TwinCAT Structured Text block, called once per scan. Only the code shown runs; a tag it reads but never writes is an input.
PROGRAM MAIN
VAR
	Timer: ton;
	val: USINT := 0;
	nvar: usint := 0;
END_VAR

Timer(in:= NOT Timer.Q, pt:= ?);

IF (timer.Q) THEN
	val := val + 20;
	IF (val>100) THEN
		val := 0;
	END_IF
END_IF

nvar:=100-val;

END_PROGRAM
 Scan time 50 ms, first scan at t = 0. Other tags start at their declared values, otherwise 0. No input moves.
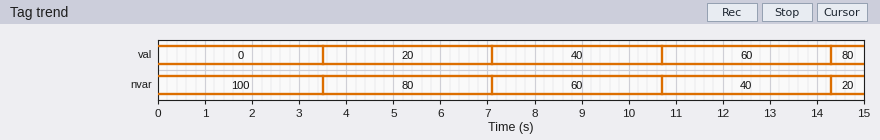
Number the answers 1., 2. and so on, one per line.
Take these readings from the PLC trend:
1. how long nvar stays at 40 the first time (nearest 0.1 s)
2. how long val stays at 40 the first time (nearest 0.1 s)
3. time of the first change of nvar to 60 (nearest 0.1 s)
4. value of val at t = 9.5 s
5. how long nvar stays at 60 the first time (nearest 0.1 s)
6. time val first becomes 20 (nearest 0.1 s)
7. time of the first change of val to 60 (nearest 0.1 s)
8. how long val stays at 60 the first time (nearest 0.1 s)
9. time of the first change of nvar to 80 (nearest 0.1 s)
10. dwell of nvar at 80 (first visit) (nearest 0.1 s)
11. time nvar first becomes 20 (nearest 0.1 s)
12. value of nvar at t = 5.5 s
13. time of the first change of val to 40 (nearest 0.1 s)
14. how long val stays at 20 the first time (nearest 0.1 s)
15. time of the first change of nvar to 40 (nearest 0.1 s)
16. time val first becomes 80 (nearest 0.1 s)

1. 3.6 s
2. 3.6 s
3. 7.1 s
4. 40
5. 3.6 s
6. 3.5 s
7. 10.7 s
8. 3.6 s
9. 3.5 s
10. 3.6 s
11. 14.3 s
12. 80
13. 7.1 s
14. 3.6 s
15. 10.7 s
16. 14.3 s
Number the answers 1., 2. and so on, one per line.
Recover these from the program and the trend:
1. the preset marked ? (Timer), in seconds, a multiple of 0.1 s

1. 3.5 s
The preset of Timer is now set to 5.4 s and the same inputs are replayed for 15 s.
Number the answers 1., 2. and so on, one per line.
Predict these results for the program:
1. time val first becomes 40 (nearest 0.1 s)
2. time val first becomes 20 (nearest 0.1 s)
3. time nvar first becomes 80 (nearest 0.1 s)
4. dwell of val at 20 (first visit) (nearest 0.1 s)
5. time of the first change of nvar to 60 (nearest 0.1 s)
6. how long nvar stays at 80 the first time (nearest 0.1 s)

1. 10.9 s
2. 5.4 s
3. 5.4 s
4. 5.5 s
5. 10.9 s
6. 5.5 s
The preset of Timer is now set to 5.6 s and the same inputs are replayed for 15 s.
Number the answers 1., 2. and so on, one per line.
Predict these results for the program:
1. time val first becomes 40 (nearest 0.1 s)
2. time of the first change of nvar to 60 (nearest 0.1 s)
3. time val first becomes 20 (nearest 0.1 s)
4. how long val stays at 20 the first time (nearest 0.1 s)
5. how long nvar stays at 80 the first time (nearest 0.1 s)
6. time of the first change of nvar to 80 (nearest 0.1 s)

1. 11.3 s
2. 11.3 s
3. 5.6 s
4. 5.7 s
5. 5.7 s
6. 5.6 s
